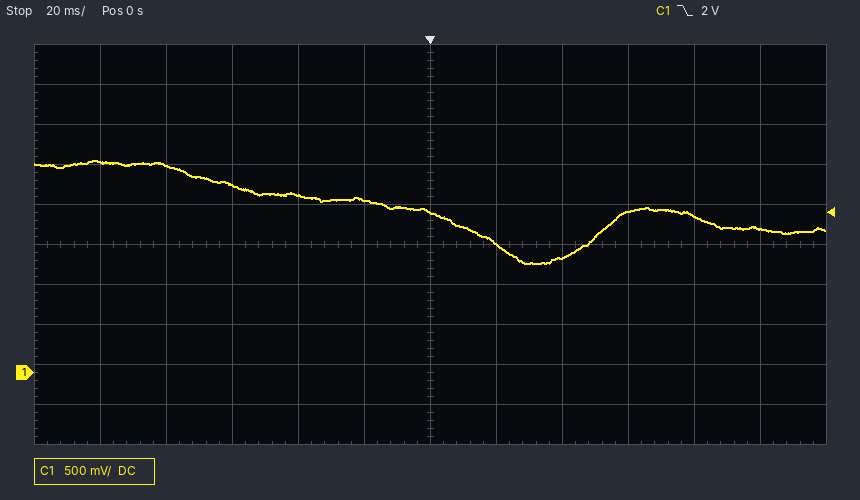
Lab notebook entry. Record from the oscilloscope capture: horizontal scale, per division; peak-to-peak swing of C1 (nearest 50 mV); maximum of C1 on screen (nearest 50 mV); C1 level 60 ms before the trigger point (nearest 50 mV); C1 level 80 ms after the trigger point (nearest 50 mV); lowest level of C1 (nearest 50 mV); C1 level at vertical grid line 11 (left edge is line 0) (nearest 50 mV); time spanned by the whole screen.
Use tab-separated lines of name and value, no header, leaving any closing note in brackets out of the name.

horizontal scale, per division	20 ms
peak-to-peak swing of C1	1.30 V
maximum of C1 on screen	2.65 V
C1 level 60 ms before the trigger point	2.35 V
C1 level 80 ms after the trigger point	1.95 V
lowest level of C1	1.35 V
C1 level at vertical grid line 11 (left edge is line 0)	1.80 V
time spanned by the whole screen	240 ms
